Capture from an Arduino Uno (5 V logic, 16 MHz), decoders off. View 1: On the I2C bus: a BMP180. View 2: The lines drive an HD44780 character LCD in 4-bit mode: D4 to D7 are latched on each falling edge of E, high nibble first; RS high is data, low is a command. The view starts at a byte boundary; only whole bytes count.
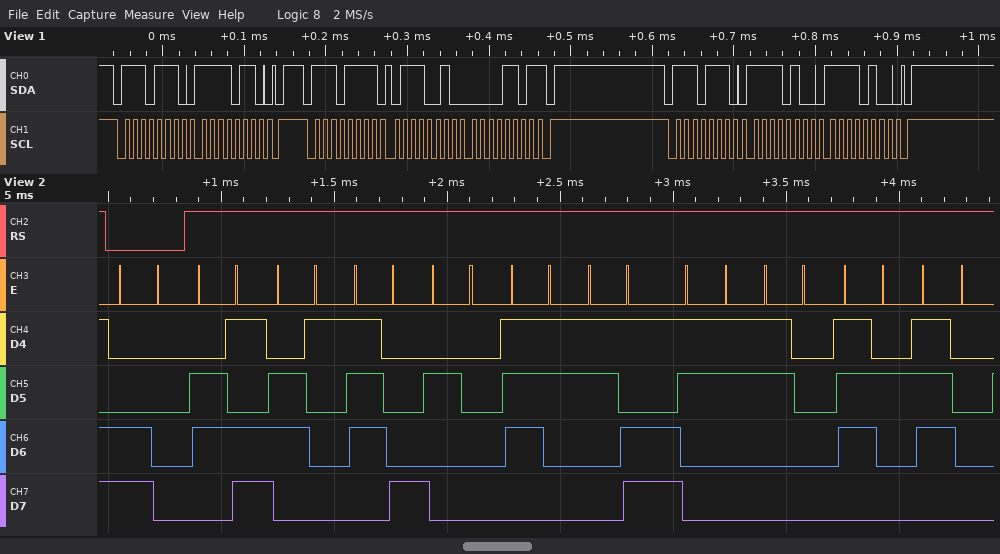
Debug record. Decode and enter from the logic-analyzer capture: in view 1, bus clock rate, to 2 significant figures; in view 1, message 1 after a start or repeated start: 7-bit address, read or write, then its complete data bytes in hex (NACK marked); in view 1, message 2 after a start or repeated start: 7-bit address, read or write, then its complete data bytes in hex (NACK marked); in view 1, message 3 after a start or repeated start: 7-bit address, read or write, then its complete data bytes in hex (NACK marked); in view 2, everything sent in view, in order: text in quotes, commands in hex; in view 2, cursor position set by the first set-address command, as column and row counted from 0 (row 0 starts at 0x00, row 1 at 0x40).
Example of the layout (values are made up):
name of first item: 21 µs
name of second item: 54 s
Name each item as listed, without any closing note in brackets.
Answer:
in view 1, bus clock rate, to 2 significant figures: 100 kHz
in view 1, message 1 after a start or repeated start: 7-bit address, read or write, then its complete data bytes in hex: 0x77 write: F6
in view 1, message 2 after a start or repeated start: 7-bit address, read or write, then its complete data bytes in hex: 0x77 read: 72 0D NACK
in view 1, message 3 after a start or repeated start: 7-bit address, read or write, then its complete data bytes in hex: 0x77 write: F4 F4
in view 2, everything sent in view, in order: text in quotes, commands in hex: 0xC0 "max s=30rp"
in view 2, cursor position set by the first set-address command, as column and row counted from 0: column 0, row 1
